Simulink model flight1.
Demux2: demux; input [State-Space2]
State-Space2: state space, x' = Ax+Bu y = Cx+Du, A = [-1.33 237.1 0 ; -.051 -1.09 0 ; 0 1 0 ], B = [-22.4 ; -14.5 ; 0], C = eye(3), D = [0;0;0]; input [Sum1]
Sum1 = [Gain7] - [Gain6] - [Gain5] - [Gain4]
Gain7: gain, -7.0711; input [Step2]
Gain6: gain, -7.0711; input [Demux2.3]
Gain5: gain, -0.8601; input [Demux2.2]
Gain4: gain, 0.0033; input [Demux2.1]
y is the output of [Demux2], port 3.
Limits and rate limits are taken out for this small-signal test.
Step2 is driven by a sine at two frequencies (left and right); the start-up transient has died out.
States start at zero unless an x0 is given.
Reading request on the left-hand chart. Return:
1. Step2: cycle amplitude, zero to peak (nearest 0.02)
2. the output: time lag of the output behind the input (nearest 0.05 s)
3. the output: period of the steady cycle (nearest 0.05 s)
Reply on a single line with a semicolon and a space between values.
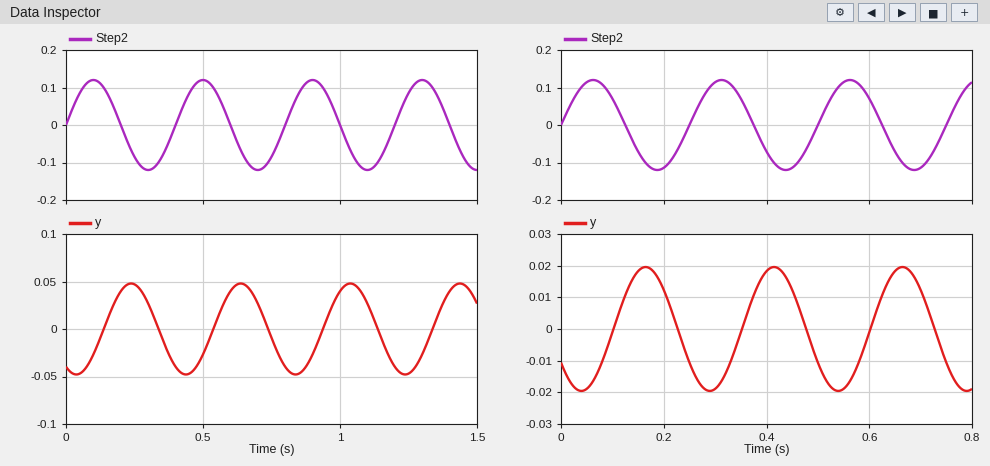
0.12; 0.15 s; 0.40 s
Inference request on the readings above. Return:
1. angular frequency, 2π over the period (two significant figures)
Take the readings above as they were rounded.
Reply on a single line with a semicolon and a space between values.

16 rad/s
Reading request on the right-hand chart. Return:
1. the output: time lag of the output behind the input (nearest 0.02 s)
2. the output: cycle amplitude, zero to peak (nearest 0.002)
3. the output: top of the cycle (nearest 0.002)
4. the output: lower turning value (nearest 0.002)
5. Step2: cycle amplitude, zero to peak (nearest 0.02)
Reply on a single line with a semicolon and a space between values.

0.10 s; 0.020; 0.020; -0.020; 0.12
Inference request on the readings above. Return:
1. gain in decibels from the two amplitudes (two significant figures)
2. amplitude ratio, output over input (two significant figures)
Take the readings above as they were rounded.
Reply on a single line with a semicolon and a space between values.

-16 dB; 0.17
